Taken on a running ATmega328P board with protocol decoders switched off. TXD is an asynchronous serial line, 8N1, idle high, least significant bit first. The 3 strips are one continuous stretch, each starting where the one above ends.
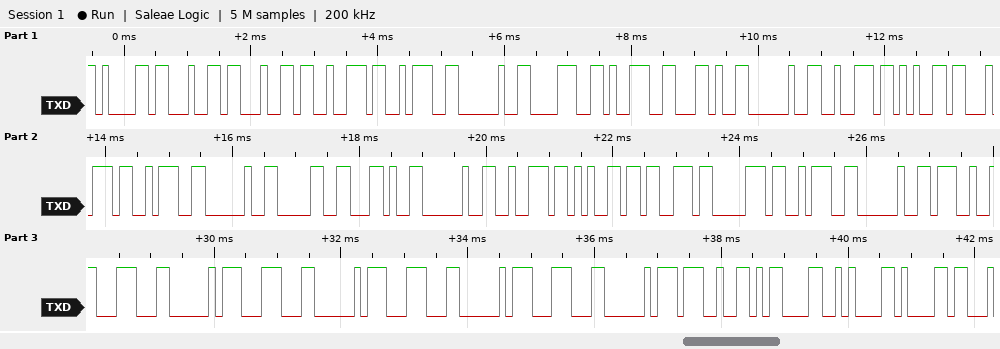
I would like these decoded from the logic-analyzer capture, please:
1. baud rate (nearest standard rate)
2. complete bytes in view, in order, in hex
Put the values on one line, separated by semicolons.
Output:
9600 baud; 61 64 64 72 3A 20 38 39 2C 20 72 65 74 3A 20 30 2C 20 72 65 73 70 3A 20 27 1C A0 1C A0 1C A0 1C A0 27 0D 0A 61
